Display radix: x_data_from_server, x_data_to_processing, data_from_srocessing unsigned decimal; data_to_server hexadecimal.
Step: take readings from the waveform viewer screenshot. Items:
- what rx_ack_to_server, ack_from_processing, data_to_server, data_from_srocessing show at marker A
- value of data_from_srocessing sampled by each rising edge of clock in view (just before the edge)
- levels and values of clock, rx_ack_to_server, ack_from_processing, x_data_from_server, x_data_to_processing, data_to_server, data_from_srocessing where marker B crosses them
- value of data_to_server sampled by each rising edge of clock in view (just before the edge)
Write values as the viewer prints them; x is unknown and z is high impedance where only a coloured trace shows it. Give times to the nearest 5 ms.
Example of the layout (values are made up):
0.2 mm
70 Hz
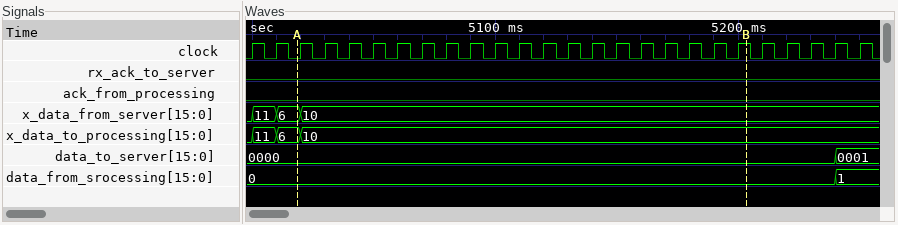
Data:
rx_ack_to_server=0, ack_from_processing=0, data_to_server=0000, data_from_srocessing=0
0, 0, 0, 0, 0, 0, 0, 0, 0, 0, 0, 0, 0, 0, 0, 0, 0, 0, 0, 0, 0, 0, 0, 0, 0, 1
clock=1, rx_ack_to_server=0, ack_from_processing=0, x_data_from_server=10, x_data_to_processing=10, data_to_server=0000, data_from_srocessing=0
0000, 0000, 0000, 0000, 0000, 0000, 0000, 0000, 0000, 0000, 0000, 0000, 0000, 0000, 0000, 0000, 0000, 0000, 0000, 0000, 0000, 0000, 0000, 0000, 0000, 0001
